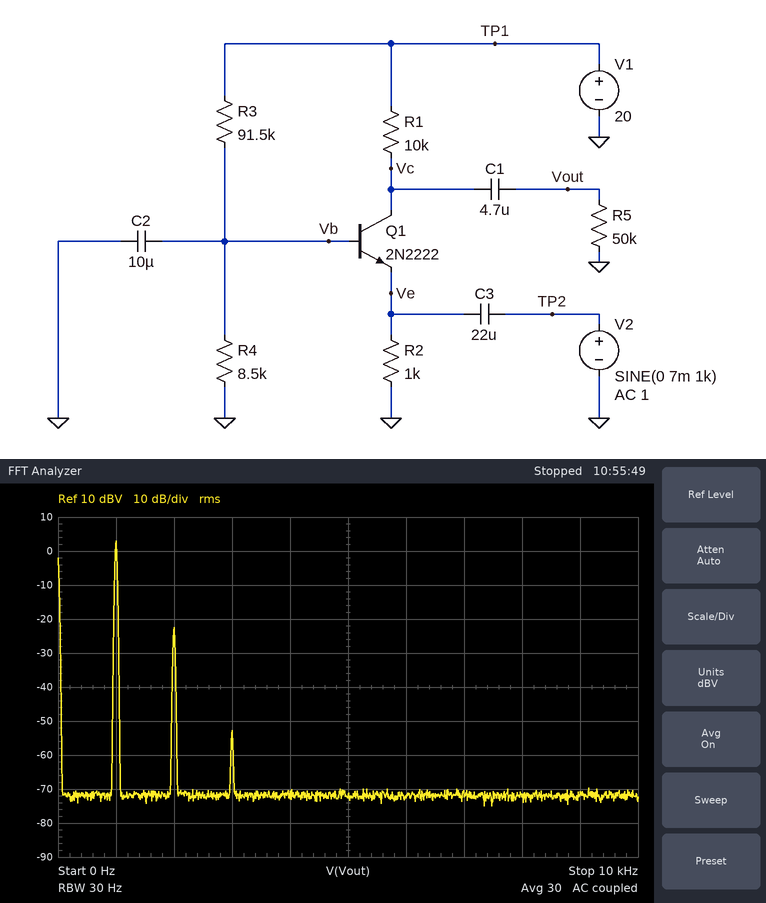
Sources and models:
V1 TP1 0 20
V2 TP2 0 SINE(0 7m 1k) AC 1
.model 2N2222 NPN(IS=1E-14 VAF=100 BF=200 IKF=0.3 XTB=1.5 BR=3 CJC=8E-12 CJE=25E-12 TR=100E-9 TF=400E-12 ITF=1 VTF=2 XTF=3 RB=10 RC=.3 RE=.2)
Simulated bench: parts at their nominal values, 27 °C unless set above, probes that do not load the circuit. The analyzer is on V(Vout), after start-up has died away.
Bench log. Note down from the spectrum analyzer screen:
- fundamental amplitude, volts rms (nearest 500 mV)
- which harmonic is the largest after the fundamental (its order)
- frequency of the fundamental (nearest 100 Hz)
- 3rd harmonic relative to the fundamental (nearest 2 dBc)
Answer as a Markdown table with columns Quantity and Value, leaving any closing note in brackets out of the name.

| Quantity | Value |
|---|---|
| fundamental amplitude, volts rms | 1.5 V |
| which harmonic is the largest after the fundamental | 2 |
| frequency of the fundamental | 1.0 kHz |
| 3rd harmonic relative to the fundamental | -56 dBc |
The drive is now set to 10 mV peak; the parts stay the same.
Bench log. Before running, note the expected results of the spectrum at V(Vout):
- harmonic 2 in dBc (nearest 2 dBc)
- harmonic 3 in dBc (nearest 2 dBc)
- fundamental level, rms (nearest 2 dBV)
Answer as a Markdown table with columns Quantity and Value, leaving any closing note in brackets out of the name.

| Quantity | Value |
|---|---|
| harmonic 2 in dBc | -22 dBc |
| harmonic 3 in dBc | -50 dBc |
| fundamental level, rms | 6 dBV |
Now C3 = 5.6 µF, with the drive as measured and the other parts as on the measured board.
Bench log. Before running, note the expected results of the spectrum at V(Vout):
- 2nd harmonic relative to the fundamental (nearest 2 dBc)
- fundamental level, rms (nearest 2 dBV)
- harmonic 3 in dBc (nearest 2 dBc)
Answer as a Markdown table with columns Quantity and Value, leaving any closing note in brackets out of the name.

| Quantity | Value |
|---|---|
| 2nd harmonic relative to the fundamental | -30 dBc |
| fundamental level, rms | 0 dBV |
| harmonic 3 in dBc | -58 dBc |
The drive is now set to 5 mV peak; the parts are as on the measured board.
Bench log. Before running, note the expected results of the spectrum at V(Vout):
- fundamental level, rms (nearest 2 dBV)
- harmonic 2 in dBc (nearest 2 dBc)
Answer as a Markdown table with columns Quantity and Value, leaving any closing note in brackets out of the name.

| Quantity | Value |
|---|---|
| fundamental level, rms | 0 dBV |
| harmonic 2 in dBc | -28 dBc |
